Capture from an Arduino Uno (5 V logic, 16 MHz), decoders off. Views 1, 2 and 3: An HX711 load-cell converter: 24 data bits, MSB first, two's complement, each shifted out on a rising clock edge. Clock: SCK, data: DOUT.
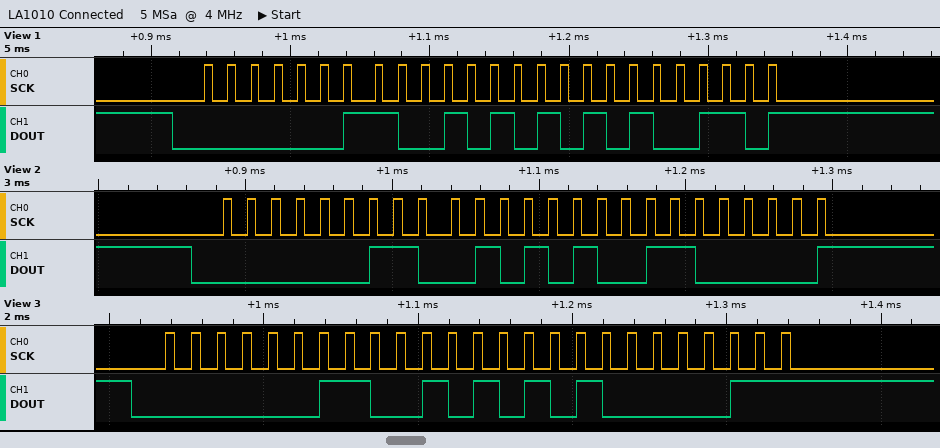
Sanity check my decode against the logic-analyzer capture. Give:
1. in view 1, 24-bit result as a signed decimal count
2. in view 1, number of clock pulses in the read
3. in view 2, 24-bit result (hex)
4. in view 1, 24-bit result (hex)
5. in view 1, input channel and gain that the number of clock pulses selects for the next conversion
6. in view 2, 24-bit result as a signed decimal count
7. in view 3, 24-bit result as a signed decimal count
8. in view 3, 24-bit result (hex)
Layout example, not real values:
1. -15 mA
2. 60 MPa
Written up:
1. 207526
2. 25
3. 0x032A60
4. 0x032AA6
5. channel A, gain 128
6. 207456
7. 207491
8. 0x032A83
